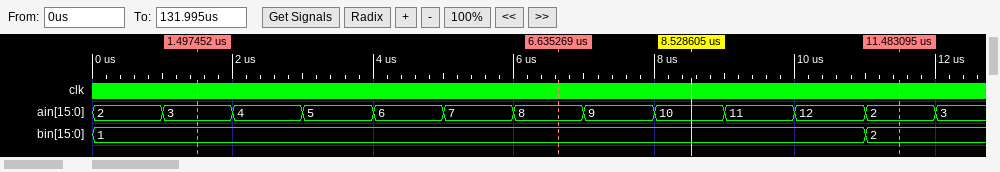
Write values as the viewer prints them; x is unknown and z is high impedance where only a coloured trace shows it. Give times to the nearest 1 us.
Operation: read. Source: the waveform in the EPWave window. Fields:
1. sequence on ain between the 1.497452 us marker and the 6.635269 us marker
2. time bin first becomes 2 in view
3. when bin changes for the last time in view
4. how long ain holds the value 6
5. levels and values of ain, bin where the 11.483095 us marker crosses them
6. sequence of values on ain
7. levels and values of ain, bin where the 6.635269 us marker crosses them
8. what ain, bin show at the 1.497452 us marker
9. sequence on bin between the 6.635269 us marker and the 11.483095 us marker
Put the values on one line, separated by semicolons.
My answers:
3, 4, 5, 6, 7, 8; 11 us; 11 us; 1 us; ain=2, bin=2; 2, 3, 4, 5, 6, 7, 8, 9, 10, 11, 12, 2, 3; ain=8, bin=1; ain=3, bin=1; 1, 2
